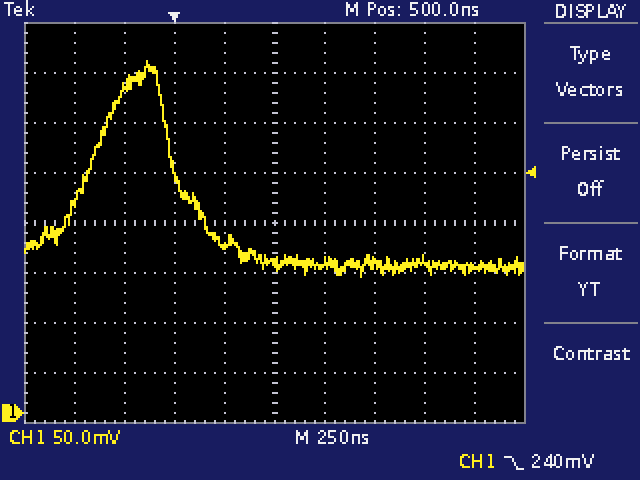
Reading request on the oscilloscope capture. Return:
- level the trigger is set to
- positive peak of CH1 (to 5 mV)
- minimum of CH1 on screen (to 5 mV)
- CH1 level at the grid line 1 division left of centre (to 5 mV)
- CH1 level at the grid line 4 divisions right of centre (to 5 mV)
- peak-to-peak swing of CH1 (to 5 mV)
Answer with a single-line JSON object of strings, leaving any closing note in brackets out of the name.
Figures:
{"level the trigger is set to": "240 mV", "positive peak of CH1": "350 mV", "minimum of CH1 on screen": "135 mV", "CH1 level at the grid line 1 division left of centre": "165 mV", "CH1 level at the grid line 4 divisions right of centre": "145 mV", "peak-to-peak swing of CH1": "215 mV"}
